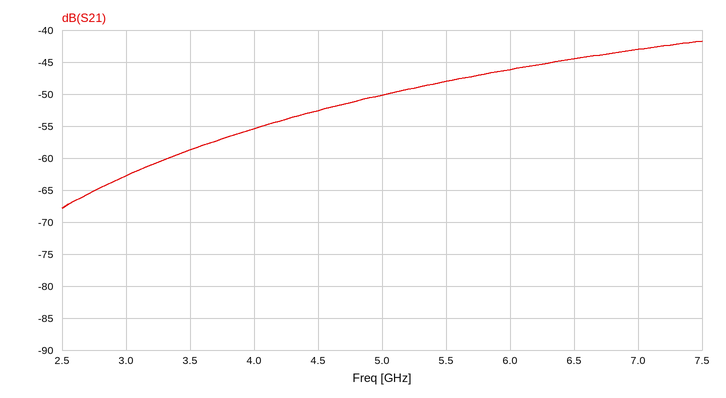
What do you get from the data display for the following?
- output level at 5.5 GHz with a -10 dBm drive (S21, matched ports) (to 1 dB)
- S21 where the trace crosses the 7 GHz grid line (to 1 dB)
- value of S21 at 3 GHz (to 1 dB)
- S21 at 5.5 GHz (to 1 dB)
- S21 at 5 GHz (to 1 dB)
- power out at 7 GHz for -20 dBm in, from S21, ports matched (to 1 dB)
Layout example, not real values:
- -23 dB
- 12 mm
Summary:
- -58 dBm
- -43 dB
- -63 dB
- -48 dB
- -50 dB
- -63 dBm
